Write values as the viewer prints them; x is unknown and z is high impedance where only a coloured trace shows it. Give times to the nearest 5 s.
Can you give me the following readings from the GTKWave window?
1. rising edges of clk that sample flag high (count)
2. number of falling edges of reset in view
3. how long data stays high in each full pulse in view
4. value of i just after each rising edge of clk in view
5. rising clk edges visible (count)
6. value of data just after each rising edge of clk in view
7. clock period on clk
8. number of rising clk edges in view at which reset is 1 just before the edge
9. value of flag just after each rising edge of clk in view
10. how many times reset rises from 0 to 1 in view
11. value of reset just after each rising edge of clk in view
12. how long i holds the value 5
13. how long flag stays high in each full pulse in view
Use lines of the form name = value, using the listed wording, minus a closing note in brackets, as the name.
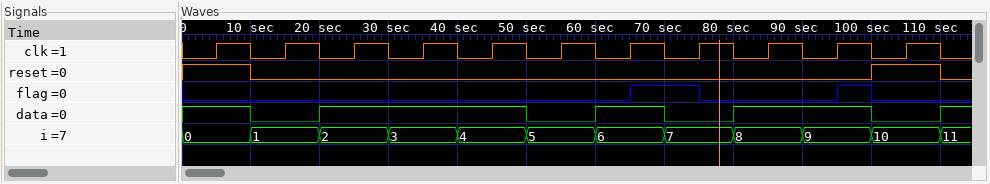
rising edges of clk that sample flag high = 1
number of falling edges of reset in view = 2
how long data stays high in each full pulse in view = 30 s, 10 s, 20 s
value of i just after each rising edge of clk in view = 0, 1, 2, 3, 4, 5, 6, 7, 8, 9, 10
rising clk edges visible = 11
value of data just after each rising edge of clk in view = 1 0 1 1 1 0 1 0 1 1 0
clock period on clk = 10 s
number of rising clk edges in view at which reset is 1 just before the edge = 2
value of flag just after each rising edge of clk in view = 0 0 0 0 0 0 1 0 0 1 0
how many times reset rises from 0 to 1 in view = 1
value of reset just after each rising edge of clk in view = 1 0 0 0 0 0 0 0 0 0 1
how long i holds the value 5 = 10 s
how long flag stays high in each full pulse in view = 10 s, 5 s
